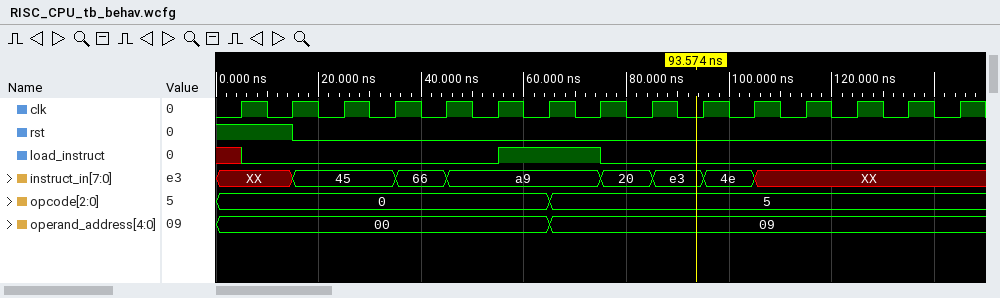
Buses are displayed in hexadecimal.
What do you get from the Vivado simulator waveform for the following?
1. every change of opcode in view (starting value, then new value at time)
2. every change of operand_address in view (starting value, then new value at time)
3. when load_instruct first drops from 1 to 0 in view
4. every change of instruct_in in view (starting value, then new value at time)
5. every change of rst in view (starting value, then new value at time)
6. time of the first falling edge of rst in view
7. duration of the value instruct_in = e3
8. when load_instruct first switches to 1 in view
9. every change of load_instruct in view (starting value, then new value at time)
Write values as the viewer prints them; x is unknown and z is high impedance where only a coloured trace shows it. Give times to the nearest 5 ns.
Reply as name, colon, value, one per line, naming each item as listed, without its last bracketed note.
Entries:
every change of opcode in view: 0, 5 at 65 ns
every change of operand_address in view: 00, 09 at 65 ns
when load_instruct first drops from 1 to 0 in view: 75 ns
every change of instruct_in in view: XX, 45 at 15 ns, 66 at 35 ns, a9 at 45 ns, 20 at 75 ns, e3 at 85 ns, 4e at 95 ns, XX at 105 ns
every change of rst in view: 1, 0 at 15 ns
time of the first falling edge of rst in view: 15 ns
duration of the value instruct_in = e3: 10 ns
when load_instruct first switches to 1 in view: 55 ns
every change of load_instruct in view: x, 0 at 5 ns, 1 at 55 ns, 0 at 75 ns
